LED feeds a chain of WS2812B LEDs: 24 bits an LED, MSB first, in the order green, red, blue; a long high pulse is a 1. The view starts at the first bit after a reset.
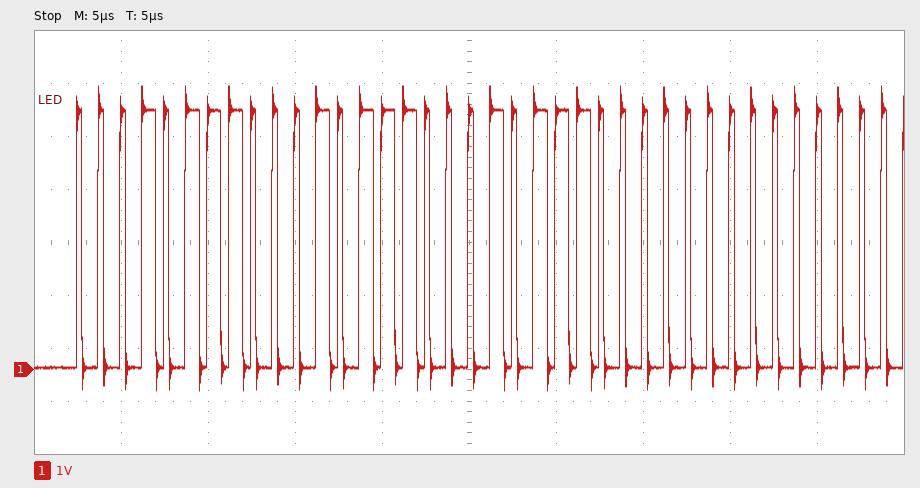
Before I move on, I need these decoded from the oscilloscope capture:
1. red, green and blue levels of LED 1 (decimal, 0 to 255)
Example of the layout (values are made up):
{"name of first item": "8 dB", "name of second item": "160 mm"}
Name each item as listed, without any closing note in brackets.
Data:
{"red, green and blue levels of LED 1": "23, 23, 23"}
